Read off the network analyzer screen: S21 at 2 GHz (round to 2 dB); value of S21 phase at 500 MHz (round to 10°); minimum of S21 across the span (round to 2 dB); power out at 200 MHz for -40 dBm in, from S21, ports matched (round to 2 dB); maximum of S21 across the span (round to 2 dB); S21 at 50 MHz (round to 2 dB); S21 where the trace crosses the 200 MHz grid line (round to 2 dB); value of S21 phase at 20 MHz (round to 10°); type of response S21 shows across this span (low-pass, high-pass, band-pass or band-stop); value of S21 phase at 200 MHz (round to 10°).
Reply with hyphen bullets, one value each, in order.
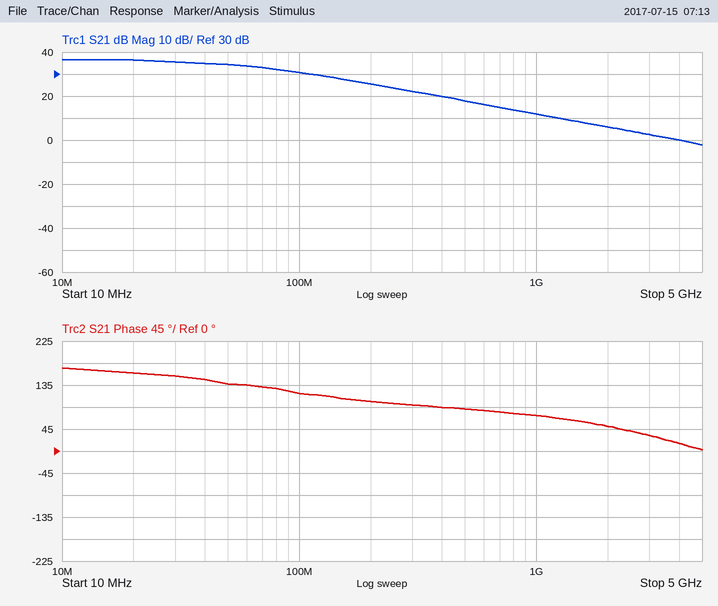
- 6 dB
- 90°
- -2 dB
- -14 dBm
- 36 dB
- 34 dB
- 26 dB
- 160°
- low-pass
- 100°
